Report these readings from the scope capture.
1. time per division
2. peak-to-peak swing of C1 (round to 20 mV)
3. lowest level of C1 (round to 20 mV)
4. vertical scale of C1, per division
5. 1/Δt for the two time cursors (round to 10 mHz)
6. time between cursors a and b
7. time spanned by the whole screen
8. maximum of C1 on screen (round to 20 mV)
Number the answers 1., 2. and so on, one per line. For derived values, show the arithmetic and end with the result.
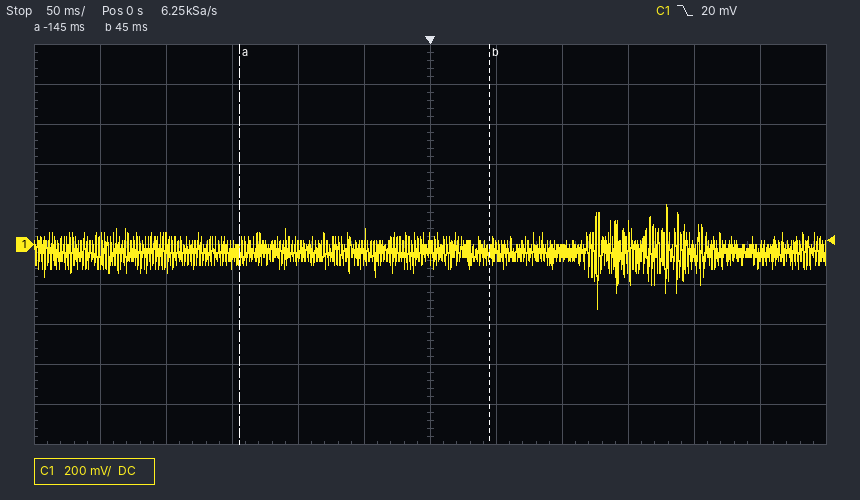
1. 50 ms
2. 200 mV − (-320 mV) = 520 mV
3. -320 mV
4. 200 mV
5. 1 / 190 ms ≈ 5.26 Hz
6. 45 ms − (-145 ms) = 190 ms
7. 600 ms
8. 200 mV
